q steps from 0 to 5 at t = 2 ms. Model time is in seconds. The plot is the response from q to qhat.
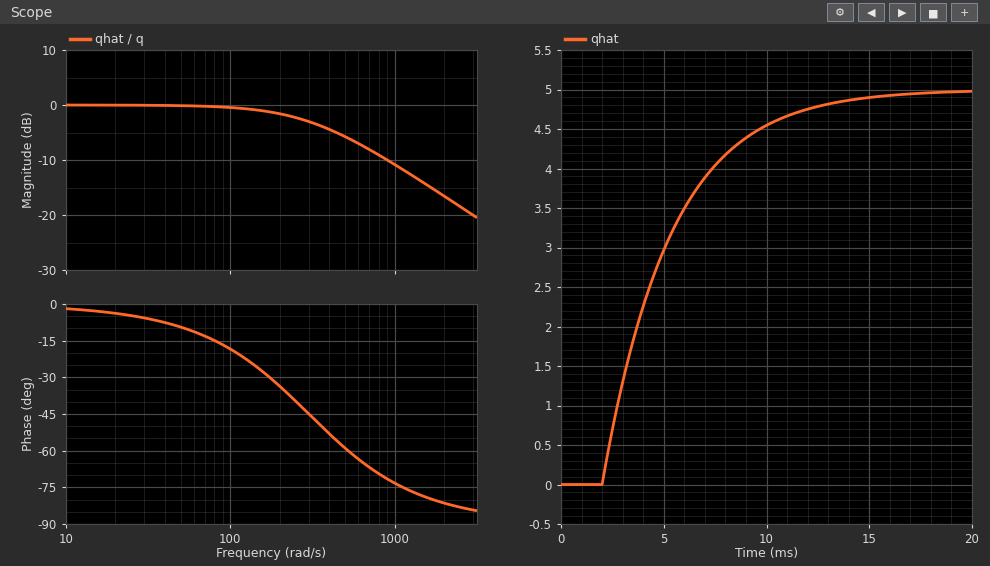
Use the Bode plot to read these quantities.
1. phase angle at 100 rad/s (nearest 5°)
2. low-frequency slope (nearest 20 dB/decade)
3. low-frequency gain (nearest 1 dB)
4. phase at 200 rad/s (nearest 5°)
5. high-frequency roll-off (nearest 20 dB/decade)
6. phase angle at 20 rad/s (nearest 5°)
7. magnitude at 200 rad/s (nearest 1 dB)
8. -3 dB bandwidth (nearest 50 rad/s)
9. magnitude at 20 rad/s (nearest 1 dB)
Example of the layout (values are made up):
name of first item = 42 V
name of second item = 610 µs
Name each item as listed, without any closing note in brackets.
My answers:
phase angle at 100 rad/s = -20°
low-frequency slope = 0 dB/decade
low-frequency gain = 0 dB
phase at 200 rad/s = -35°
high-frequency roll-off = -20 dB/decade
phase angle at 20 rad/s = -5°
magnitude at 200 rad/s = -2 dB
-3 dB bandwidth = 300 rad/s
magnitude at 20 rad/s = 0 dB
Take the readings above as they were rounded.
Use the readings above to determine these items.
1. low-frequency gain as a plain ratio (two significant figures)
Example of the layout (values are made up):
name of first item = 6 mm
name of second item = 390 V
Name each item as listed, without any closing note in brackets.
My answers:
low-frequency gain as a plain ratio = 1.0
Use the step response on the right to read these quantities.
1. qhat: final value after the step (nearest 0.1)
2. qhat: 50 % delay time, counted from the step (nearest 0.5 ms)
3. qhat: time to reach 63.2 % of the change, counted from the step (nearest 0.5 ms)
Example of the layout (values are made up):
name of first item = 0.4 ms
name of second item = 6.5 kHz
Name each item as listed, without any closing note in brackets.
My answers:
qhat: final value after the step = 5.0
qhat: 50 % delay time, counted from the step = 2.5 ms
qhat: time to reach 63.2 % of the change, counted from the step = 3.5 ms
